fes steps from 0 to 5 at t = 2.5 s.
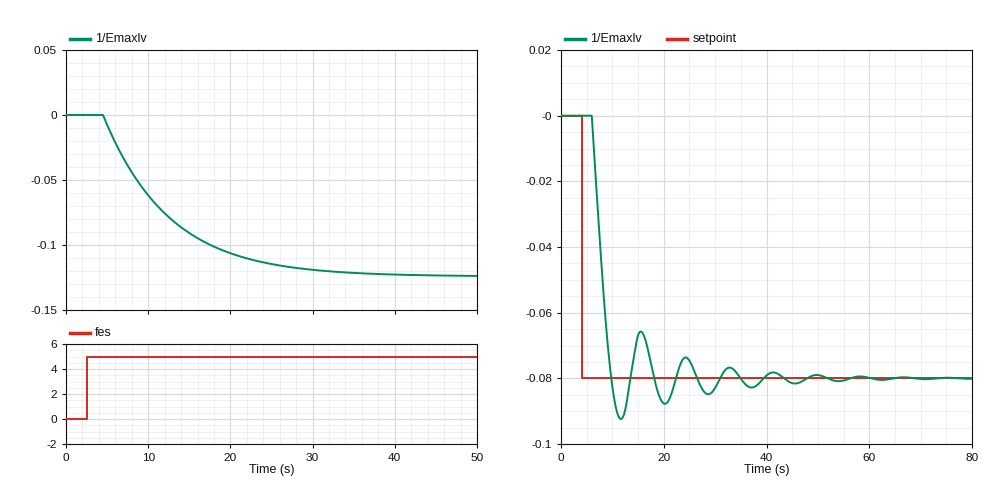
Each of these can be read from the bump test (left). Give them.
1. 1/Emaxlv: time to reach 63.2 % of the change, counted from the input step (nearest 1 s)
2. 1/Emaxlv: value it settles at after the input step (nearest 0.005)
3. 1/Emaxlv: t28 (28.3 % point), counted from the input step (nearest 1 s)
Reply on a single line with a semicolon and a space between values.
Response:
10 s; -0.125; 5 s
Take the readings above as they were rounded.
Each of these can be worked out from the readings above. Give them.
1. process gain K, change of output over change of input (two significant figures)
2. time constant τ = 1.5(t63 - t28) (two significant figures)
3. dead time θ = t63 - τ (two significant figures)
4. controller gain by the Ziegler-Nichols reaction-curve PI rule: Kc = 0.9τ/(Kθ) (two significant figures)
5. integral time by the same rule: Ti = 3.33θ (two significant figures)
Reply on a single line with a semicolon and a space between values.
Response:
-0.025; 7.5 s; 2.5 s; -110; 8.3 s
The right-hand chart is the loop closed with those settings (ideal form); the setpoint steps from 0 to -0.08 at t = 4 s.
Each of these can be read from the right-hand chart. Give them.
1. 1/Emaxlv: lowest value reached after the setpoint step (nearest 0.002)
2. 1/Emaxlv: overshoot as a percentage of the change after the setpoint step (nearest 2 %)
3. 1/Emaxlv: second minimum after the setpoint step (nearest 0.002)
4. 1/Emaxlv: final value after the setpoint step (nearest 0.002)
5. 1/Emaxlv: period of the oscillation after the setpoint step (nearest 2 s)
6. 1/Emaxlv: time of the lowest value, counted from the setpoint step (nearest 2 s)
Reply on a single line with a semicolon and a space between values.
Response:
-0.092; 16 %; -0.088; -0.080; 8 s; 8 s
